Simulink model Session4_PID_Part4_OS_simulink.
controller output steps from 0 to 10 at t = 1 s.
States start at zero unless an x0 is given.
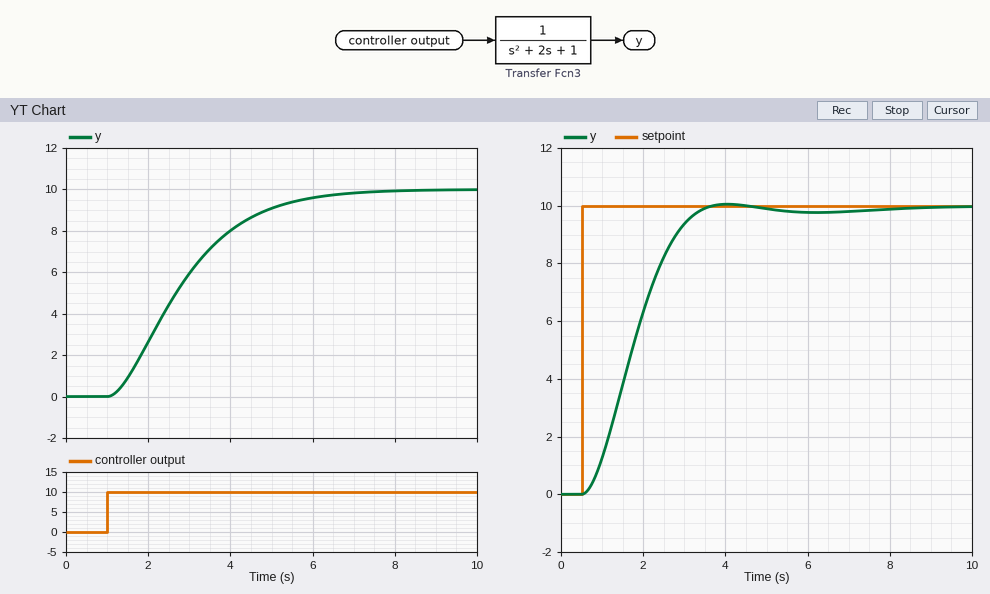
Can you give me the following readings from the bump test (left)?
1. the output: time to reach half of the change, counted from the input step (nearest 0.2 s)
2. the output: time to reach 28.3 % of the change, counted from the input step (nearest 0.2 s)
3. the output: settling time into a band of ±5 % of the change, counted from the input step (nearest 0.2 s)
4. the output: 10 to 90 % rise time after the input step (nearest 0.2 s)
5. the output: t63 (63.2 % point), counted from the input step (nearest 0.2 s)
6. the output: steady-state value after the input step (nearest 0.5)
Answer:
1.6 s
1.0 s
4.8 s
3.4 s
2.2 s
10.0
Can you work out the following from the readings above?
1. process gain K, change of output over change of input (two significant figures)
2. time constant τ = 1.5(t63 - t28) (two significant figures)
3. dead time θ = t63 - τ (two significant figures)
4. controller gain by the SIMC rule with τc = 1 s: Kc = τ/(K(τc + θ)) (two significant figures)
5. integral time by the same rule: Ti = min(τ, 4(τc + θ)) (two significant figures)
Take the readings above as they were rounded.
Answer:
1.0
1.8 s
0.40 s
1.3
1.8 s
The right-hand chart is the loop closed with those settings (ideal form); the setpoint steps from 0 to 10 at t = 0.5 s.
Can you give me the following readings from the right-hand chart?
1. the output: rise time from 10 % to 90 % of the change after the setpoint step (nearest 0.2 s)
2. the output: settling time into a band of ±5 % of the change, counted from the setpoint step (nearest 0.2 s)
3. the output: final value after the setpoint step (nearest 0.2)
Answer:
1.8 s
2.6 s
10.0
